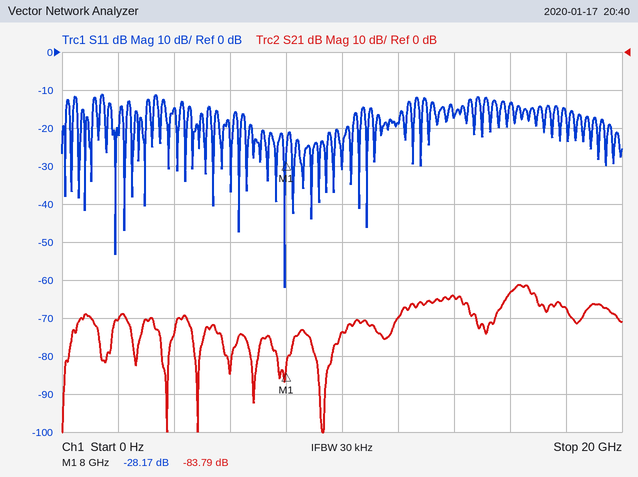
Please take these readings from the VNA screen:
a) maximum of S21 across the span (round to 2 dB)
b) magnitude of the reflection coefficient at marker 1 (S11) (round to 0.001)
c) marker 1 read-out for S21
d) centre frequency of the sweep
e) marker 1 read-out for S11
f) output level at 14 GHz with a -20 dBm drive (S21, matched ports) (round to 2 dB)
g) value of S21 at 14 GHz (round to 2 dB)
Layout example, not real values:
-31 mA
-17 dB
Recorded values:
-62 dB
0.039
-83.79 dB
10 GHz
-28.17 dB
-84 dBm
-64 dB
